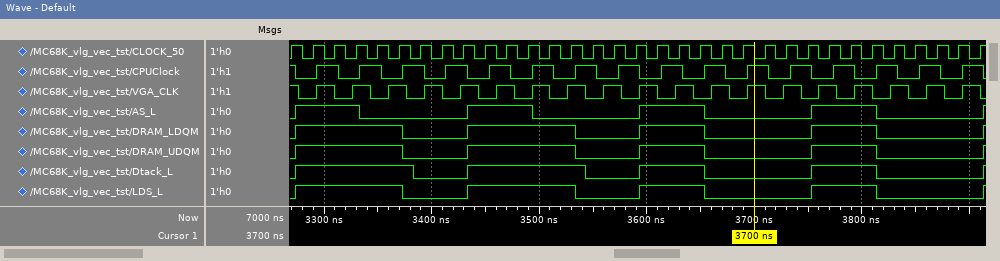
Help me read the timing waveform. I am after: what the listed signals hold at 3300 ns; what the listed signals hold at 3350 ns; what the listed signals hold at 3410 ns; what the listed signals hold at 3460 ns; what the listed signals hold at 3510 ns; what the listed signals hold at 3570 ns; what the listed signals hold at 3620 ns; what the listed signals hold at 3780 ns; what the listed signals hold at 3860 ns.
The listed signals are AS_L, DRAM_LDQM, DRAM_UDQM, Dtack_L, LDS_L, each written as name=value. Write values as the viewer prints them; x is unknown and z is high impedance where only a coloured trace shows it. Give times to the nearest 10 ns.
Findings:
AS_L=1, DRAM_LDQM=1, DRAM_UDQM=1, Dtack_L=1, LDS_L=1
AS_L=0, DRAM_LDQM=1, DRAM_UDQM=1, Dtack_L=1, LDS_L=1
AS_L=0, DRAM_LDQM=0, DRAM_UDQM=0, Dtack_L=0, LDS_L=0
AS_L=1, DRAM_LDQM=1, DRAM_UDQM=1, Dtack_L=1, LDS_L=1
AS_L=0, DRAM_LDQM=1, DRAM_UDQM=1, Dtack_L=1, LDS_L=1
AS_L=0, DRAM_LDQM=0, DRAM_UDQM=0, Dtack_L=0, LDS_L=0
AS_L=1, DRAM_LDQM=1, DRAM_UDQM=1, Dtack_L=1, LDS_L=1
AS_L=1, DRAM_LDQM=1, DRAM_UDQM=1, Dtack_L=1, LDS_L=1
AS_L=0, DRAM_LDQM=0, DRAM_UDQM=0, Dtack_L=0, LDS_L=0
